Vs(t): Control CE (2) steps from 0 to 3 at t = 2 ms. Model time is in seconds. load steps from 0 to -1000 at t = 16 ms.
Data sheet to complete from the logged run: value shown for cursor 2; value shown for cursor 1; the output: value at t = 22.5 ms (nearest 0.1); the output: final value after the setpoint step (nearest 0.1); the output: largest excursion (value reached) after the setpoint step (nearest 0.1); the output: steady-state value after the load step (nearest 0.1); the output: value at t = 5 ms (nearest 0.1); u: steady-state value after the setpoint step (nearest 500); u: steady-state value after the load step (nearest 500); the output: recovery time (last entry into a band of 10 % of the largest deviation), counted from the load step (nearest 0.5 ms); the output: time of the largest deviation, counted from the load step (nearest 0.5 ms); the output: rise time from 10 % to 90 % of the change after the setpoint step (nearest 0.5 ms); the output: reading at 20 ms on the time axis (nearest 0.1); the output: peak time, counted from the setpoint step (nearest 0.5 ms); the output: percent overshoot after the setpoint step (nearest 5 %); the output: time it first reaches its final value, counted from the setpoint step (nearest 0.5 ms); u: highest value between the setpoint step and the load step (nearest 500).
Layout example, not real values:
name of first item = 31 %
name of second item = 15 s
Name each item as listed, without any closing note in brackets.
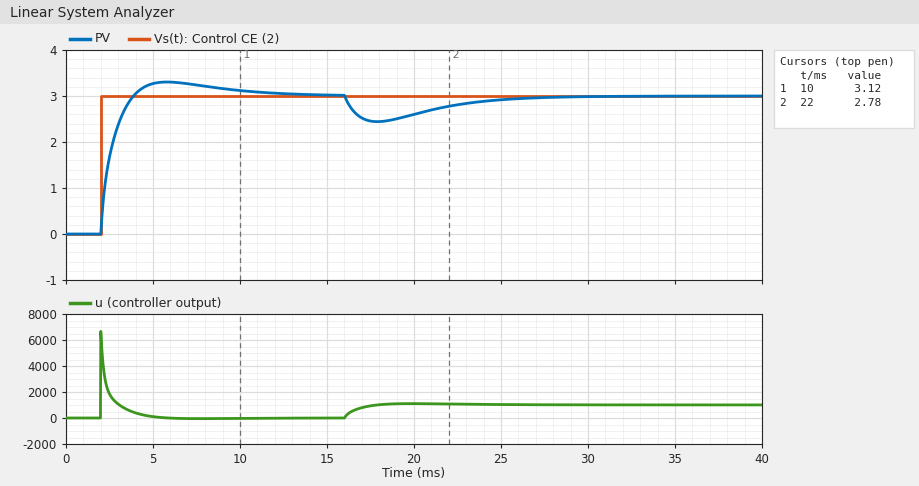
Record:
value shown for cursor 2 = 2.78
value shown for cursor 1 = 3.12
the output: value at t = 22.5 ms = 2.8
the output: final value after the setpoint step = 3.0
the output: largest excursion (value reached) after the setpoint step = 3.3
the output: steady-state value after the load step = 3.0
the output: value at t = 5 ms = 3.3
u: steady-state value after the setpoint step = 0
u: steady-state value after the load step = 1000
the output: recovery time (last entry into a band of 10 % of the largest deviation), counted from the load step = 10.0 ms
the output: time of the largest deviation, counted from the load step = 2.0 ms
the output: rise time from 10 % to 90 % of the change after the setpoint step = 1.5 ms
the output: reading at 20 ms on the time axis = 2.6
the output: peak time, counted from the setpoint step = 4.0 ms
the output: percent overshoot after the setpoint step = 10 %
the output: time it first reaches its final value, counted from the setpoint step = 2.0 ms
u: highest value between the setpoint step and the load step = 6500
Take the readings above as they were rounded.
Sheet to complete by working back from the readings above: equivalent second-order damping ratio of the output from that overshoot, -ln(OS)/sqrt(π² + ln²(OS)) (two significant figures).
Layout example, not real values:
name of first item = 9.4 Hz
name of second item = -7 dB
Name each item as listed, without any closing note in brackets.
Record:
equivalent second-order damping ratio of the output from that overshoot, -ln(OS)/sqrt(π² + ln²(OS)) = 0.59
